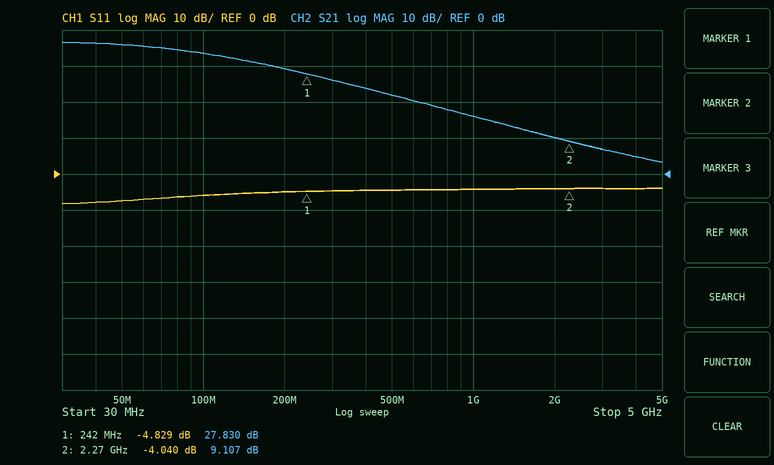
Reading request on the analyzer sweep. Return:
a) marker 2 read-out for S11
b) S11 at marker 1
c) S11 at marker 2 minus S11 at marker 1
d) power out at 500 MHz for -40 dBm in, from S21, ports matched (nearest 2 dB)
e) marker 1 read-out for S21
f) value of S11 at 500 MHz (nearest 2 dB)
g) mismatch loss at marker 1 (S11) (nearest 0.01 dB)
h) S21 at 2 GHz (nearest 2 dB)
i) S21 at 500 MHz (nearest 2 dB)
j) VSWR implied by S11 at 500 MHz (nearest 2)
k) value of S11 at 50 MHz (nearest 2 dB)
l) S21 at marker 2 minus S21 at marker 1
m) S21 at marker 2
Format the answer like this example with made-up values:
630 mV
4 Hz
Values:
-4.040 dB
-4.829 dB
0.789 dB
-18 dBm
27.830 dB
-4 dB
1.73 dB
10 dB
22 dB
4
-8 dB
-18.723 dB
9.107 dB
